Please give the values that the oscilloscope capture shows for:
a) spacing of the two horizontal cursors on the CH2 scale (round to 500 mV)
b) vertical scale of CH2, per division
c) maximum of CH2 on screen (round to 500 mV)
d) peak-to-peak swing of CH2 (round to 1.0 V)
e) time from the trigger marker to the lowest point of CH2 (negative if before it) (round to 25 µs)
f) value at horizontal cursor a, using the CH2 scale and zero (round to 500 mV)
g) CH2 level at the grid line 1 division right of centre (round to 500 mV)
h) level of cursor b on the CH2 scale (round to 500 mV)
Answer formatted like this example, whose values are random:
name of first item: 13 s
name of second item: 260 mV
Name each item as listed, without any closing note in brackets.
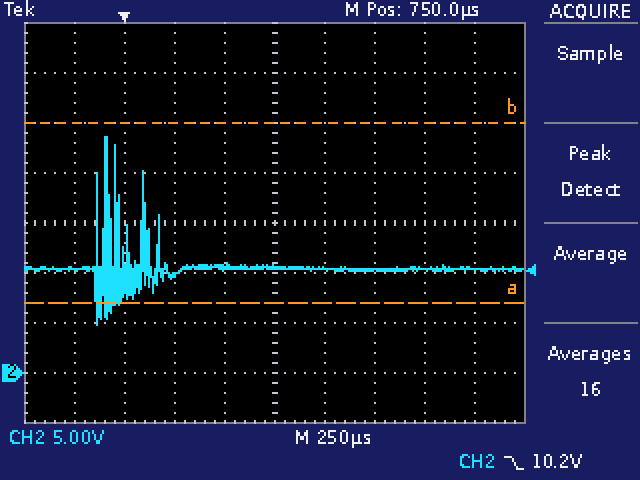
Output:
spacing of the two horizontal cursors on the CH2 scale: 18.0 V
vertical scale of CH2, per division: 5 V
maximum of CH2 on screen: 23.5 V
peak-to-peak swing of CH2: 19.0 V
time from the trigger marker to the lowest point of CH2 (negative if before it): -125 µs
value at horizontal cursor a, using the CH2 scale and zero: 7.0 V
CH2 level at the grid line 1 division right of centre: 10.5 V
level of cursor b on the CH2 scale: 25.0 V
